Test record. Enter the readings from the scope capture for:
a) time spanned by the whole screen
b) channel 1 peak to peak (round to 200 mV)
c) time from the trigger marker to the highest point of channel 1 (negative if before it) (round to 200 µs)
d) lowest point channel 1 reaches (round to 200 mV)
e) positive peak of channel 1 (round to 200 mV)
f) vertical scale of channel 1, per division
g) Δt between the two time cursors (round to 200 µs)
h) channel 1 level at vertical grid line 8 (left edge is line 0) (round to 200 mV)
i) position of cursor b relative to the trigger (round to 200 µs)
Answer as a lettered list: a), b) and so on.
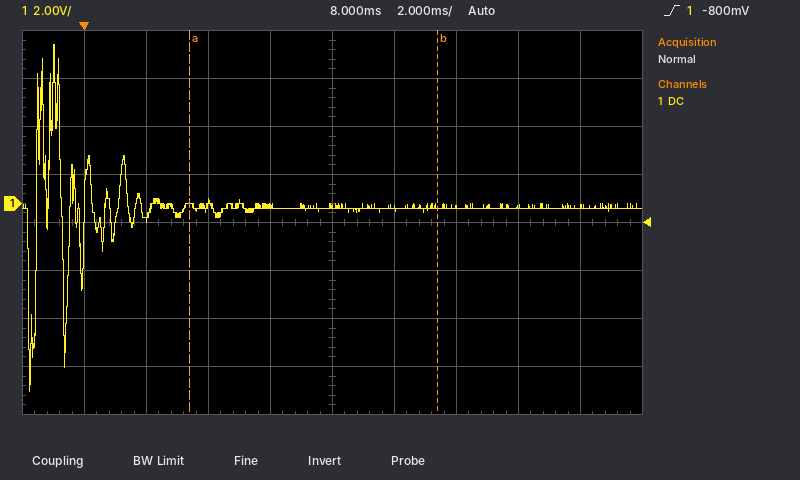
a) 20 ms
b) 14.4 V
c) -1.0 ms
d) -7.8 V
e) 6.6 V
f) 2 V
g) 8.0 ms
h) -200 mV
i) +11.4 ms
